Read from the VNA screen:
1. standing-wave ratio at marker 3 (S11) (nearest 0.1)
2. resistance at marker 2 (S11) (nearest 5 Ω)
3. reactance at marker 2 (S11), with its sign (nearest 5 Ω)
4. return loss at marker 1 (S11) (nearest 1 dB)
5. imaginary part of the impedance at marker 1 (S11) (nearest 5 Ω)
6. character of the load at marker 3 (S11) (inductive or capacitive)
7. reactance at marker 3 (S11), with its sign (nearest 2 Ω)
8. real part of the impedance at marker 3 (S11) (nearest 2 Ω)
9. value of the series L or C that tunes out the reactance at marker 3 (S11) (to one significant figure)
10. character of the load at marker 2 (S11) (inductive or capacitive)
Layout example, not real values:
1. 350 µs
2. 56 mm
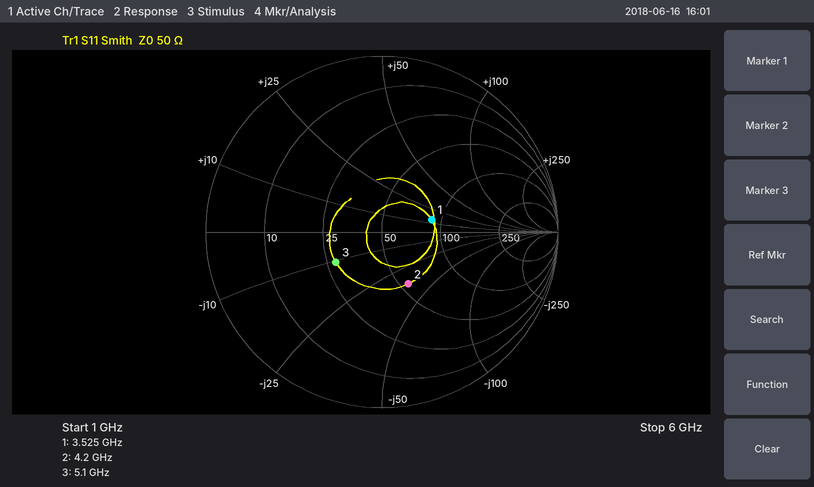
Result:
1. 1.9
2. 55 Ω
3. -35 Ω
4. 11 dB
5. +15 Ω
6. capacitive
7. -10 Ω
8. 28 Ω
9. 300 pH
10. capacitive
